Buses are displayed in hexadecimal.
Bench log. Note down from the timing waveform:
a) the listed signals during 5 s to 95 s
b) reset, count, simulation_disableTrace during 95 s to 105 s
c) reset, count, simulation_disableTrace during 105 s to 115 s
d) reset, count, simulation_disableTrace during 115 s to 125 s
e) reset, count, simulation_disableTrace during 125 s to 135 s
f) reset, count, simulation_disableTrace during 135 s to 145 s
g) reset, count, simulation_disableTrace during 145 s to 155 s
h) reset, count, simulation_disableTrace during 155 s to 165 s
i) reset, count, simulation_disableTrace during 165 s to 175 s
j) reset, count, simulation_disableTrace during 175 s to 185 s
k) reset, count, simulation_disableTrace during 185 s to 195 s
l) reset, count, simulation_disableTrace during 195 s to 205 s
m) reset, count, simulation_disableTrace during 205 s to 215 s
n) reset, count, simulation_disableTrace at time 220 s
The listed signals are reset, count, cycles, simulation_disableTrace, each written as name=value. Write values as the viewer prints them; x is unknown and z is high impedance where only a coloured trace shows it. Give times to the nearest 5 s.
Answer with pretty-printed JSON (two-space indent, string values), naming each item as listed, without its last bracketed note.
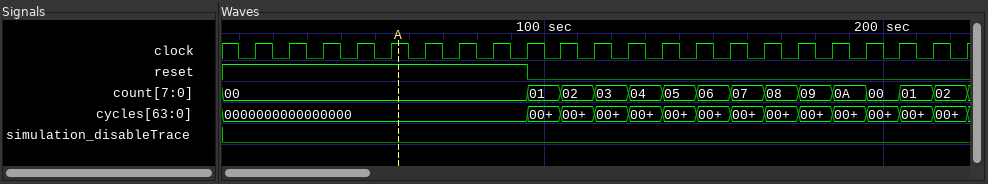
{
  "the listed signals during 5 s to 95 s": "reset=1, count=00, cycles=0000000000000000, simulation_disableTrace=0",
  "reset, count, simulation_disableTrace during 95 s to 105 s": "reset=0, count=01, simulation_disableTrace=0",
  "reset, count, simulation_disableTrace during 105 s to 115 s": "reset=0, count=02, simulation_disableTrace=0",
  "reset, count, simulation_disableTrace during 115 s to 125 s": "reset=0, count=03, simulation_disableTrace=0",
  "reset, count, simulation_disableTrace during 125 s to 135 s": "reset=0, count=04, simulation_disableTrace=0",
  "reset, count, simulation_disableTrace during 135 s to 145 s": "reset=0, count=05, simulation_disableTrace=0",
  "reset, count, simulation_disableTrace during 145 s to 155 s": "reset=0, count=06, simulation_disableTrace=0",
  "reset, count, simulation_disableTrace during 155 s to 165 s": "reset=0, count=07, simulation_disableTrace=0",
  "reset, count, simulation_disableTrace during 165 s to 175 s": "reset=0, count=08, simulation_disableTrace=0",
  "reset, count, simulation_disableTrace during 175 s to 185 s": "reset=0, count=09, simulation_disableTrace=0",
  "reset, count, simulation_disableTrace during 185 s to 195 s": "reset=0, count=0A, simulation_disableTrace=0",
  "reset, count, simulation_disableTrace during 195 s to 205 s": "reset=0, count=00, simulation_disableTrace=0",
  "reset, count, simulation_disableTrace during 205 s to 215 s": "reset=0, count=01, simulation_disableTrace=0",
  "reset, count, simulation_disableTrace at time 220 s": "reset=0, count=02, simulation_disableTrace=0"
}
